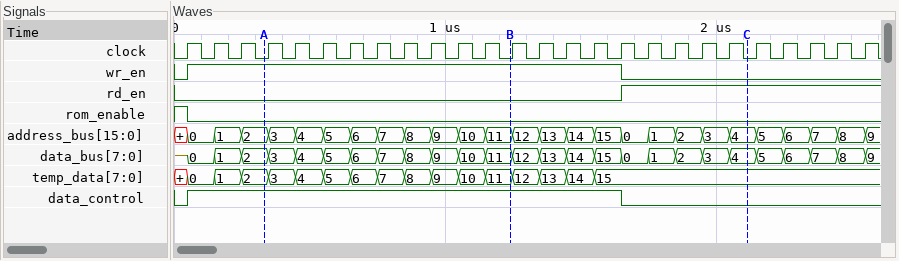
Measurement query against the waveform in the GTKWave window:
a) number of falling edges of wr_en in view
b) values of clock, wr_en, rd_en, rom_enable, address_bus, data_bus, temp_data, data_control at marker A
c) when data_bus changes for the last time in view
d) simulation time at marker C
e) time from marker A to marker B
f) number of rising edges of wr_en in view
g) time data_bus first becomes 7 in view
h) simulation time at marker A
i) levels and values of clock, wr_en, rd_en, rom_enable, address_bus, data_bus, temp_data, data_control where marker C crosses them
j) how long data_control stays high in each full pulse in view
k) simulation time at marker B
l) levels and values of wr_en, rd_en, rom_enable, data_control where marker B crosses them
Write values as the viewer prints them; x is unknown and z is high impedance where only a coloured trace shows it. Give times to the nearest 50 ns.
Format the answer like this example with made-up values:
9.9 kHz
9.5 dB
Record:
1
clock=0, wr_en=1, rd_en=0, rom_enable=0, address_bus=2, data_bus=2, temp_data=2, data_control=1
2550 ns
2100 ns
900 ns
1
750 ns
350 ns
clock=0, wr_en=0, rd_en=1, rom_enable=0, address_bus=4, data_bus=4, temp_data=15, data_control=0
1600 ns
1250 ns
wr_en=1, rd_en=0, rom_enable=0, data_control=1
